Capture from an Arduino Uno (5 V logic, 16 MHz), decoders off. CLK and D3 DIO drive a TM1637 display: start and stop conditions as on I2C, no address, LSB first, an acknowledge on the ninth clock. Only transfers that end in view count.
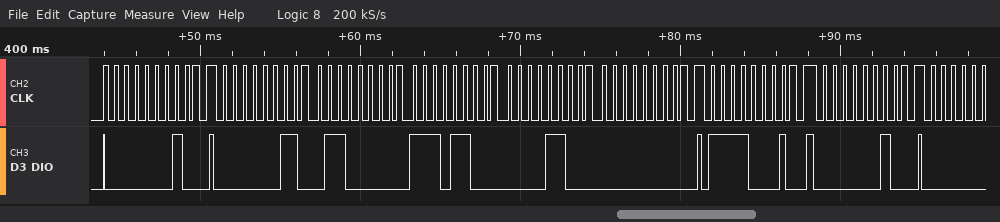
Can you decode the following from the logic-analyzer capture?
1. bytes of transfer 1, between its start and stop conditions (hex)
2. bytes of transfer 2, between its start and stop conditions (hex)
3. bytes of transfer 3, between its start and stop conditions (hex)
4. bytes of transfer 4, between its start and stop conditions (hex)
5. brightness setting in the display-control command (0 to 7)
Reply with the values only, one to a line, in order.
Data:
40
C0 06 37 30 00
8F
40
7
